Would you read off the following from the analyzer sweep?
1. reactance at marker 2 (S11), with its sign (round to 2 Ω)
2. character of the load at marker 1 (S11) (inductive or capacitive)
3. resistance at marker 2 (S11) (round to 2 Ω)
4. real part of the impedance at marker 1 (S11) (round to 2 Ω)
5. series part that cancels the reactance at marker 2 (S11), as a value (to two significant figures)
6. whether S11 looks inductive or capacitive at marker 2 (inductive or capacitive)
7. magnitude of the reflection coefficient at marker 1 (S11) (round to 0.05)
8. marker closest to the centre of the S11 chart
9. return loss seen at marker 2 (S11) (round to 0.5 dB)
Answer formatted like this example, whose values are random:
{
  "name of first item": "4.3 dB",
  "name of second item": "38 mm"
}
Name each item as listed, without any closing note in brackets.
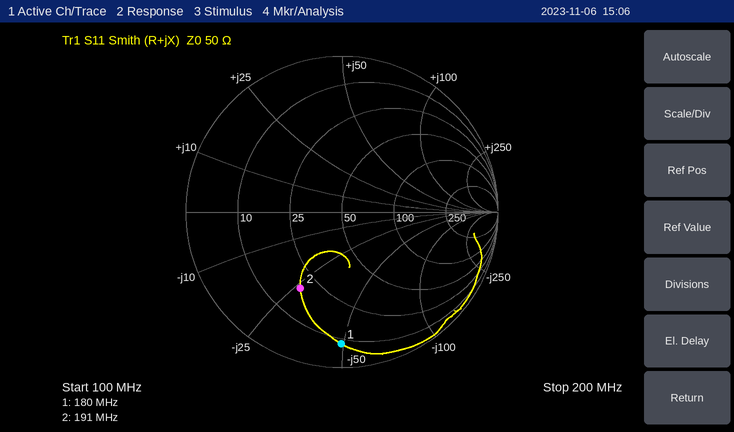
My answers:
{
  "reactance at marker 2 (S11), with its sign": "-26 Ω",
  "character of the load at marker 1 (S11)": "capacitive",
  "resistance at marker 2 (S11)": "18 Ω",
  "real part of the impedance at marker 1 (S11)": "8 Ω",
  "series part that cancels the reactance at marker 2 (S11), as a value": "22 nH",
  "whether S11 looks inductive or capacitive at marker 2": "capacitive",
  "magnitude of the reflection coefficient at marker 1 (S11)": "0.85",
  "marker closest to the centre of the S11 chart": "marker 2",
  "return loss seen at marker 2 (S11)": "5.0 dB"
}
